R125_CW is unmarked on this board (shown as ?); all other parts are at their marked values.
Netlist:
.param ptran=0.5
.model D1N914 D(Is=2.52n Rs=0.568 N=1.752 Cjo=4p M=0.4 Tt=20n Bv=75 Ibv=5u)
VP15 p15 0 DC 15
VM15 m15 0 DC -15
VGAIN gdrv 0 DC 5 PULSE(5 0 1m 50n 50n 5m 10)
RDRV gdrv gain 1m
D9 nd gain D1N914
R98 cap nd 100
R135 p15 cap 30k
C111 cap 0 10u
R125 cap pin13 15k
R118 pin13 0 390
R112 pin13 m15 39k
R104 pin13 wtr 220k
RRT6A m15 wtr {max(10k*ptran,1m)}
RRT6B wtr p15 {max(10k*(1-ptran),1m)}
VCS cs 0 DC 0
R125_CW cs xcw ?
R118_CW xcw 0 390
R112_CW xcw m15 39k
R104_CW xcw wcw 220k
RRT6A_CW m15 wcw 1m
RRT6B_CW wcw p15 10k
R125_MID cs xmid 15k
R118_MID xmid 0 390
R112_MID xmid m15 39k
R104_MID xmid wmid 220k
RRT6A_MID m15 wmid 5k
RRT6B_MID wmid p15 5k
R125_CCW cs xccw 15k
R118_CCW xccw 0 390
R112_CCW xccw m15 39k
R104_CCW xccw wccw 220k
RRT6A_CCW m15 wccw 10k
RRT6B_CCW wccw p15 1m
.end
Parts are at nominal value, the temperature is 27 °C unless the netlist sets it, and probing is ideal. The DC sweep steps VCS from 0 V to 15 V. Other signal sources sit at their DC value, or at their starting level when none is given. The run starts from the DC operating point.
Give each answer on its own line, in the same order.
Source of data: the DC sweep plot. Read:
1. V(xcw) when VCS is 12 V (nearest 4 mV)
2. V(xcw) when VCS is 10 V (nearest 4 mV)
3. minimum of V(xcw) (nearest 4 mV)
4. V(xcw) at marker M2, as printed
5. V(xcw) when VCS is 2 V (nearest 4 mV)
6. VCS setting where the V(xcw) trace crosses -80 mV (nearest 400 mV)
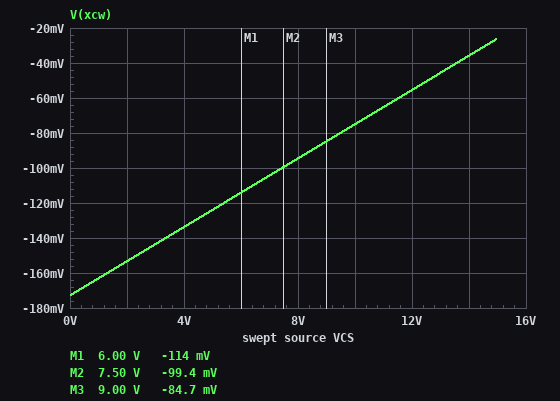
-56 mV
-76 mV
-172 mV
-99.4 mV
-152 mV
9.6 V
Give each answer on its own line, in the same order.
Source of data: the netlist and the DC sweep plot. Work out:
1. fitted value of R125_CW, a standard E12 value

39 kΩ
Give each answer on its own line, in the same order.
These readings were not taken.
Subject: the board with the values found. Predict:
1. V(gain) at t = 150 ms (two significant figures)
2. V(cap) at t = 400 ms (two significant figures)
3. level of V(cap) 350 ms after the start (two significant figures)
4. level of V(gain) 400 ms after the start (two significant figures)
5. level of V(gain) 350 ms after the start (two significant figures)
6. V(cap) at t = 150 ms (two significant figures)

5.0 V
4.9 V
4.8 V
5.0 V
5.0 V
3.9 V
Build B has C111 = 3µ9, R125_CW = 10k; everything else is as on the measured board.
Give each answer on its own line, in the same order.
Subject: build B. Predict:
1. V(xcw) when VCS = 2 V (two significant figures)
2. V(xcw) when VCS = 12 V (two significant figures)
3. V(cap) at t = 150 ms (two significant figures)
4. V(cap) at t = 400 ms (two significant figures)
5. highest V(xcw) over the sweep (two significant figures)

-94 mV
280 mV
4.9 V
5.0 V
390 mV
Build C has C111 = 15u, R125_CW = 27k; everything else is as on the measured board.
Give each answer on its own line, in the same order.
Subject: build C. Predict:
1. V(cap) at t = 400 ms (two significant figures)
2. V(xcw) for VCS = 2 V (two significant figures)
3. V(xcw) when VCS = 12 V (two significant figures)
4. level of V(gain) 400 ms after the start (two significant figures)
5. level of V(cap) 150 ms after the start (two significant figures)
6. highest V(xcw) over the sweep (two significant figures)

4.7 V
-140 mV
-3.2 mV
5.0 V
3.4 V
39 mV
